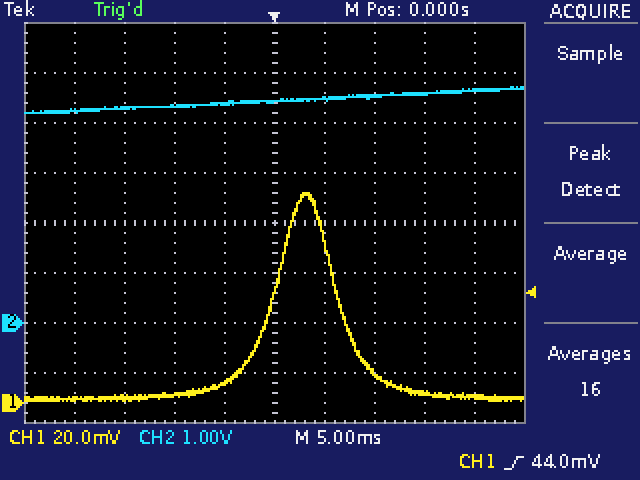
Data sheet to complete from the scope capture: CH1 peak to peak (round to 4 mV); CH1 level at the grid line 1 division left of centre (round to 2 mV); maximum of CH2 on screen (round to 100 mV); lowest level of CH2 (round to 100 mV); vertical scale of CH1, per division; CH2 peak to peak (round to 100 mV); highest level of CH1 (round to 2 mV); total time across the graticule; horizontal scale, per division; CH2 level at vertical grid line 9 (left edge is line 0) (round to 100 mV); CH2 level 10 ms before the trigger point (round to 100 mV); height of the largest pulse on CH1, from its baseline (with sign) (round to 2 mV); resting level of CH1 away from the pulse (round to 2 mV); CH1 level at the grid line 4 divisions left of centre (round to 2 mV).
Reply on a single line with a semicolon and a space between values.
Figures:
84 mV; 8 mV; 4.7 V; 4.2 V; 20 mV; 500 mV; 84 mV; 50 ms; 5 ms; 4.7 V; 4.3 V; +82 mV; 2 mV; 2 mV
